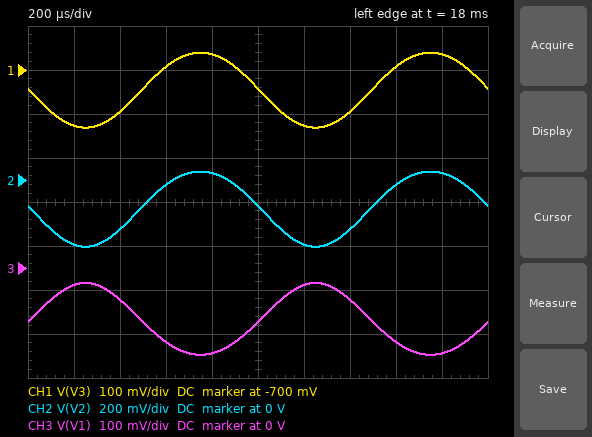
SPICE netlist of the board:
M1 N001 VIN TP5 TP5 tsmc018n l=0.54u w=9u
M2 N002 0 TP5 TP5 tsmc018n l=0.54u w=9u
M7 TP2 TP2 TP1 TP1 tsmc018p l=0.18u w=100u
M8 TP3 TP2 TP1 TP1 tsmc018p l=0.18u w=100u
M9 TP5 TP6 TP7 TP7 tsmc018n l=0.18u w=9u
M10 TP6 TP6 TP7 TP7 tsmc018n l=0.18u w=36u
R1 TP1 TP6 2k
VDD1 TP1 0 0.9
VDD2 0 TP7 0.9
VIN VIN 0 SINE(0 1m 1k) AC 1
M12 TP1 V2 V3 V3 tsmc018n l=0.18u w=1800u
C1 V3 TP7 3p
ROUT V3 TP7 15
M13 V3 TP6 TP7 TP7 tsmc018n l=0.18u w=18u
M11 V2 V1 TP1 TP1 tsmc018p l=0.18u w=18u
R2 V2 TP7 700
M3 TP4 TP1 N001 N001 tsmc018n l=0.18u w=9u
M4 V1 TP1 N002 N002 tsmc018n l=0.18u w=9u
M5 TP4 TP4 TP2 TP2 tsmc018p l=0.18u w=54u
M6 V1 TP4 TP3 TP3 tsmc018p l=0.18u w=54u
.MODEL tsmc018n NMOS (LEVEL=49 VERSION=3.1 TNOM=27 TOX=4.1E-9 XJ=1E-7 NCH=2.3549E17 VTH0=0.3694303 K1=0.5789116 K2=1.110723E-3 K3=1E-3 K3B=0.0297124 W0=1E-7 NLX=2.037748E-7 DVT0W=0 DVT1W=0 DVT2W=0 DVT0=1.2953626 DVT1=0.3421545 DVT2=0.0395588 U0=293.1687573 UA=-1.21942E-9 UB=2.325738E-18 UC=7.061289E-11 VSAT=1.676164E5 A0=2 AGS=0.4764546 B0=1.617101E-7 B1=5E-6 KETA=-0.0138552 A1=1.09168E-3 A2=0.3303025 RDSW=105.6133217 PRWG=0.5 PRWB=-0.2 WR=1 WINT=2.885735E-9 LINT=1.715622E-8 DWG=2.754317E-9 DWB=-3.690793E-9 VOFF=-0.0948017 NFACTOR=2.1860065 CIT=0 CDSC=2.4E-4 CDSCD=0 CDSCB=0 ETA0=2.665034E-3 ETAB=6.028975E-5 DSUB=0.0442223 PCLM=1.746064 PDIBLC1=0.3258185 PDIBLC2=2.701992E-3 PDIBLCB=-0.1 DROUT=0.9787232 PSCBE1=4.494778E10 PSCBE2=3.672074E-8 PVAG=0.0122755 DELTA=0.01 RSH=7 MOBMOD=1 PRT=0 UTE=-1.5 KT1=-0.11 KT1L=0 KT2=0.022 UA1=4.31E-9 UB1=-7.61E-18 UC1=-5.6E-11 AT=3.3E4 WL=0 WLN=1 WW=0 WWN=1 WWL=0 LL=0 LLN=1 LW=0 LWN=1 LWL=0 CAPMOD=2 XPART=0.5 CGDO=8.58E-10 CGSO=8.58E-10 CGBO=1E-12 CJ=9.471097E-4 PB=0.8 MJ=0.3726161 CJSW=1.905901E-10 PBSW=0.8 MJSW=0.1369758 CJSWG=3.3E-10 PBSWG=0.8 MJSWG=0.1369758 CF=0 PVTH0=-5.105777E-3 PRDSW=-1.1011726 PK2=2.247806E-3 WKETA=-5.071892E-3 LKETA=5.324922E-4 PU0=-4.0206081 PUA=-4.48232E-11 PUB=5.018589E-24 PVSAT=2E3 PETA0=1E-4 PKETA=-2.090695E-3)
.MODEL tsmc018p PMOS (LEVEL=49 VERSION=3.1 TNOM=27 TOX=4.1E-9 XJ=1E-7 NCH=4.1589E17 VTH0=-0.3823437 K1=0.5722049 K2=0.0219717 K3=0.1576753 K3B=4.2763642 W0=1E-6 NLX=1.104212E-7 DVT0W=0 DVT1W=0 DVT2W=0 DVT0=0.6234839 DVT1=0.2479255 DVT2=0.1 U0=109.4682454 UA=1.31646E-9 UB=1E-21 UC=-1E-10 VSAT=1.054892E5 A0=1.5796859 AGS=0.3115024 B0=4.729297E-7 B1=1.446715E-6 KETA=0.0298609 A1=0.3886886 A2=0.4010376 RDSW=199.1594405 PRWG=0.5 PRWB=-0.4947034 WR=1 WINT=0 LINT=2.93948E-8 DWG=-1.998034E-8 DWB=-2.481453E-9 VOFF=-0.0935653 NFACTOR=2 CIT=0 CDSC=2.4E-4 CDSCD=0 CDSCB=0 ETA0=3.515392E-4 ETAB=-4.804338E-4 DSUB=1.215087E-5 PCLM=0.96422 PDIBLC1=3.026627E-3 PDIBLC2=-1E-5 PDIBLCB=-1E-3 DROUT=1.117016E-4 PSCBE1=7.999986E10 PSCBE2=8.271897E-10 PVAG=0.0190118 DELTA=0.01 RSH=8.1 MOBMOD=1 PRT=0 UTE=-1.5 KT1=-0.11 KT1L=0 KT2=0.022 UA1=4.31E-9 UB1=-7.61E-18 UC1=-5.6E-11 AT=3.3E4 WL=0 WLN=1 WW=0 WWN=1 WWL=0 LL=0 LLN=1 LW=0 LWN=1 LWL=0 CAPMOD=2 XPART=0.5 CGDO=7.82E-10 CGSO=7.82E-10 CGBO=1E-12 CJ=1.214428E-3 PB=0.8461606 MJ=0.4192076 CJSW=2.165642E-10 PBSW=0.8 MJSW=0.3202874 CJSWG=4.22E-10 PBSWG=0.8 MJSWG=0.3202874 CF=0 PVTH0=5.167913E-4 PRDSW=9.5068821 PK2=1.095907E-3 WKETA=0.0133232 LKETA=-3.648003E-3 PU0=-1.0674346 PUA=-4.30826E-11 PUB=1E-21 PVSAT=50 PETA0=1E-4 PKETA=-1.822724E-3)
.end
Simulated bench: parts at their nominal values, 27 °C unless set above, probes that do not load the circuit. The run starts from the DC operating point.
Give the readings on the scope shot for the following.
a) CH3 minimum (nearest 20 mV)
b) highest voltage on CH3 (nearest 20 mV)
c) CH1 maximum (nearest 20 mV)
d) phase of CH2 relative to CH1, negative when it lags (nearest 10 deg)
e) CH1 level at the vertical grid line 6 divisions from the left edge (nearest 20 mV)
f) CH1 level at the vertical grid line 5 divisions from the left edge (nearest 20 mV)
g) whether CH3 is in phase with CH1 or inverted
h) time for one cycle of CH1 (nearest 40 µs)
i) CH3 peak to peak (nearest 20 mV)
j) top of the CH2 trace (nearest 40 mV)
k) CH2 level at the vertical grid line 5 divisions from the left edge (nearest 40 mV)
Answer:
-200 mV
-40 mV
-660 mV
0 deg
-820 mV
-740 mV
inverted
1.00 ms
160 mV
40 mV
-120 mV
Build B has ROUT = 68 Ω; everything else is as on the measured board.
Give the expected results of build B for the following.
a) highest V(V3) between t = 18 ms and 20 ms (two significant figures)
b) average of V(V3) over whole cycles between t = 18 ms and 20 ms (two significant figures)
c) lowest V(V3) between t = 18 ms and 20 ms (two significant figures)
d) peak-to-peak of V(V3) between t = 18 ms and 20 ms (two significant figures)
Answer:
-520 mV
-640 mV
-770 mV
250 mV
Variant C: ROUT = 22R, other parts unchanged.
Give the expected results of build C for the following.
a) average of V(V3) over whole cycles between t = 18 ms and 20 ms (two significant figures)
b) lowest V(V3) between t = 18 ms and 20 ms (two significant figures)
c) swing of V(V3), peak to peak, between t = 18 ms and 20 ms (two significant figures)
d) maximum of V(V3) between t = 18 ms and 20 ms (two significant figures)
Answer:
-720 mV
-820 mV
200 mV
-620 mV
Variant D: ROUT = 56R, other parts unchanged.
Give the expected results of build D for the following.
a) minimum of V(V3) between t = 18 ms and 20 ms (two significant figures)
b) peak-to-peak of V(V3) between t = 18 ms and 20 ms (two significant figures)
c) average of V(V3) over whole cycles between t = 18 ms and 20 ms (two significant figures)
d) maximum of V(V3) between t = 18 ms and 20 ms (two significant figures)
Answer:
-780 mV
250 mV
-650 mV
-530 mV
